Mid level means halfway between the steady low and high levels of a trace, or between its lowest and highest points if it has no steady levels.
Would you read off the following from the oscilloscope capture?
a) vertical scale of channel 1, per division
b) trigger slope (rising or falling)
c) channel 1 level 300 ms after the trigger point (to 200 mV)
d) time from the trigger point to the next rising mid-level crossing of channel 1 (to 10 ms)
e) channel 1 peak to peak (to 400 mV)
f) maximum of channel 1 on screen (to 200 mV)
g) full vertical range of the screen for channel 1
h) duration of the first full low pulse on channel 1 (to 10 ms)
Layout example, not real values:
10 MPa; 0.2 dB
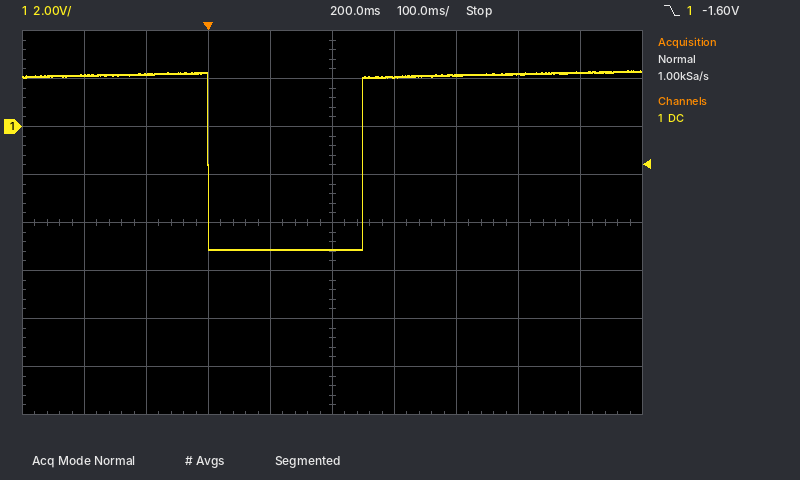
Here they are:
2 V; falling; 2.0 V; 250 ms; 7.6 V; 2.4 V; 16 V; 250 ms
